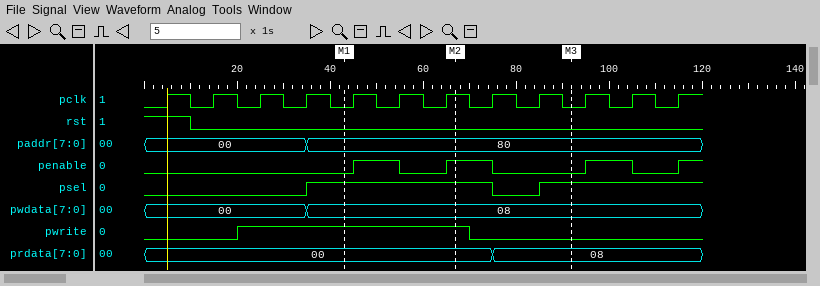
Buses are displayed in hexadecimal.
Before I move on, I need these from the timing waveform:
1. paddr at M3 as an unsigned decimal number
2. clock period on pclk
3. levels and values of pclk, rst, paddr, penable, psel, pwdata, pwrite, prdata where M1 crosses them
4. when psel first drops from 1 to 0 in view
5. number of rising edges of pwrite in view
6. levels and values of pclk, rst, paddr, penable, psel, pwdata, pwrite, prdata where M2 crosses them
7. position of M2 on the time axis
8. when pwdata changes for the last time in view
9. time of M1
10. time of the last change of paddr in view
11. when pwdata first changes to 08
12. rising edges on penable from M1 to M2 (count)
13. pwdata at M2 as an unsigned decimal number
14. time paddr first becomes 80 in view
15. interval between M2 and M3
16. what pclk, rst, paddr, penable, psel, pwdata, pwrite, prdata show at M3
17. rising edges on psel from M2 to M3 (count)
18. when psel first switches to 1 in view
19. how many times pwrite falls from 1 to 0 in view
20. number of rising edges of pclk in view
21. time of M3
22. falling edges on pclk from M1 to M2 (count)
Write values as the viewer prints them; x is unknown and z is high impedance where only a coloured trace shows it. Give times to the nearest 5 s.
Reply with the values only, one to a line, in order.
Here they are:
128
10 s
pclk=0, rst=0, paddr=80, penable=0, psel=1, pwdata=08, pwrite=1, prdata=00
75 s
1
pclk=1, rst=0, paddr=80, penable=1, psel=1, pwdata=08, pwrite=1, prdata=00
65 s
35 s
45 s
35 s
35 s
2
8
35 s
25 s
pclk=0, rst=0, paddr=80, penable=0, psel=1, pwdata=08, pwrite=0, prdata=08
1
35 s
1
12
90 s
2
